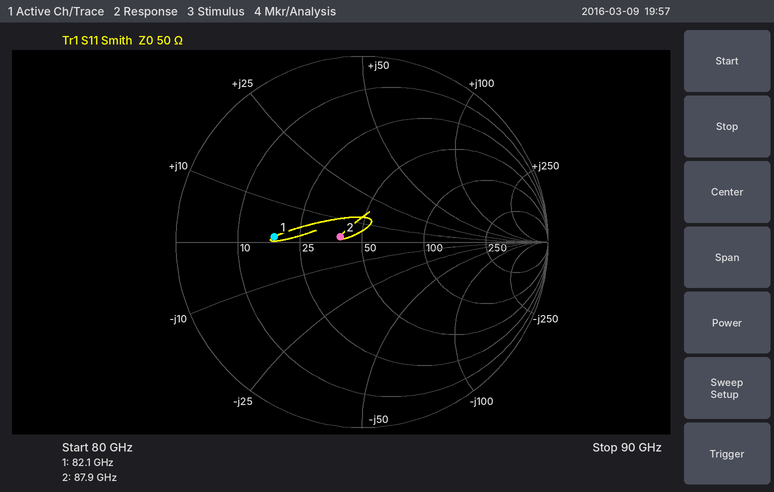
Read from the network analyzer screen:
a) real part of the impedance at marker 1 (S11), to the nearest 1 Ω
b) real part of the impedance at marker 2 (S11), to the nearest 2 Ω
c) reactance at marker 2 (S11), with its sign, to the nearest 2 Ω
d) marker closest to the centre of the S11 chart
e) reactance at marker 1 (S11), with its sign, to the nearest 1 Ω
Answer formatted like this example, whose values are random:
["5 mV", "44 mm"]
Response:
["18 Ω", "40 Ω", "+2 Ω", "marker 2", "+1 Ω"]
